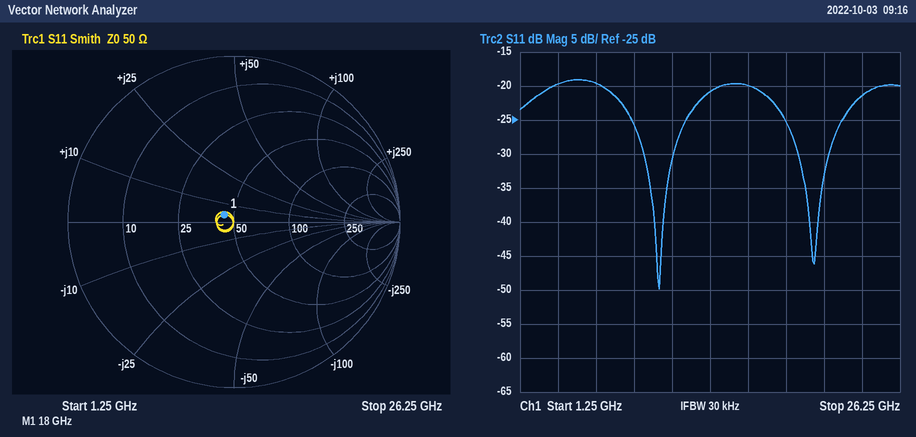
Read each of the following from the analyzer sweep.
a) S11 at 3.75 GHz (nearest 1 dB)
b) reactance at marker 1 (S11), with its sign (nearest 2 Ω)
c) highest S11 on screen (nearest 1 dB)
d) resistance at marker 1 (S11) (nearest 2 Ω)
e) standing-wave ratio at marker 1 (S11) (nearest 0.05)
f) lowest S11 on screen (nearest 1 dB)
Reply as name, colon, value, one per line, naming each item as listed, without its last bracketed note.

S11 at 3.75 GHz: -20 dB
reactance at marker 1 (S11), with its sign: +4 Ω
highest S11 on screen: -19 dB
resistance at marker 1 (S11): 44 Ω
standing-wave ratio at marker 1 (S11): 1.15
lowest S11 on screen: -50 dB
